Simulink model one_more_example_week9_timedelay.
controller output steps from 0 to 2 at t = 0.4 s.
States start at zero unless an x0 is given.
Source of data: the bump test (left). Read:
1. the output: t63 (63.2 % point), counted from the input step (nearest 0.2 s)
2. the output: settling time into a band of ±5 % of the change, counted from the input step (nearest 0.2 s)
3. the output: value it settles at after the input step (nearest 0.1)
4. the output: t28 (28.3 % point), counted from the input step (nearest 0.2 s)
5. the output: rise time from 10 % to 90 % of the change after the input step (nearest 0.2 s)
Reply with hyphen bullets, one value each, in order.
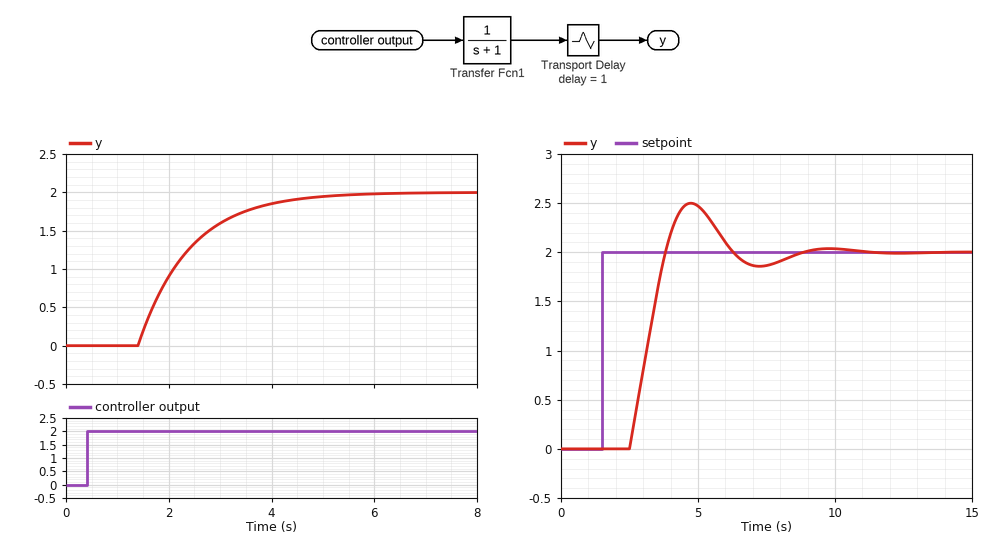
- 2.0 s
- 4.0 s
- 2.0
- 1.4 s
- 2.2 s
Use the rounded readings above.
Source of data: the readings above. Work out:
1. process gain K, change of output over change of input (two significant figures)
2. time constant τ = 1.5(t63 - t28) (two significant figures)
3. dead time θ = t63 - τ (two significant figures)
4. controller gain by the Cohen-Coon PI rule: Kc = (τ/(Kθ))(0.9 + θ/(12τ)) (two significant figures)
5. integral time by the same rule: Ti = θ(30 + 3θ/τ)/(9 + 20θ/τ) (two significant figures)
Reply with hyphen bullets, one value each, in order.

- 1.0
- 0.90 s
- 1.1 s
- 0.82
- 1.1 s
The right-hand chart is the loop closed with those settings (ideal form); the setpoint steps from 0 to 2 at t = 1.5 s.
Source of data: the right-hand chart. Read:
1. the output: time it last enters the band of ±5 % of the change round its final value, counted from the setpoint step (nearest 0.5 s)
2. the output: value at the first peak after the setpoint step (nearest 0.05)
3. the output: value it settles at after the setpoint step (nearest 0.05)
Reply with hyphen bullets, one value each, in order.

- 6.5 s
- 2.50
- 2.00
